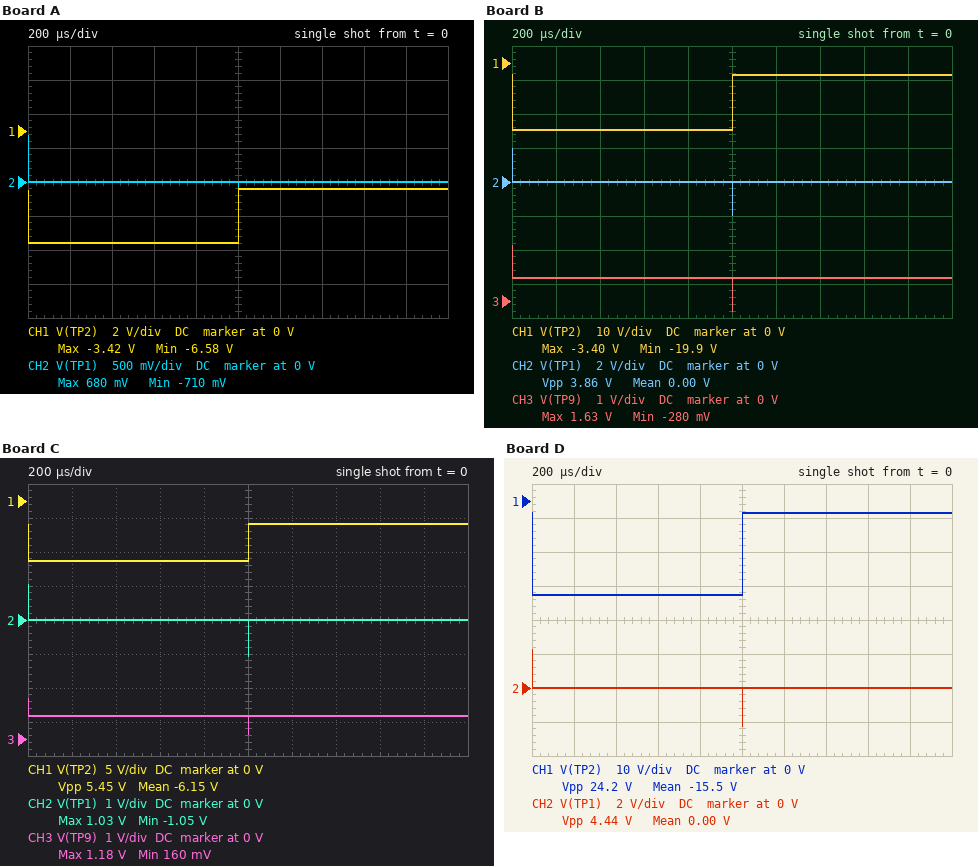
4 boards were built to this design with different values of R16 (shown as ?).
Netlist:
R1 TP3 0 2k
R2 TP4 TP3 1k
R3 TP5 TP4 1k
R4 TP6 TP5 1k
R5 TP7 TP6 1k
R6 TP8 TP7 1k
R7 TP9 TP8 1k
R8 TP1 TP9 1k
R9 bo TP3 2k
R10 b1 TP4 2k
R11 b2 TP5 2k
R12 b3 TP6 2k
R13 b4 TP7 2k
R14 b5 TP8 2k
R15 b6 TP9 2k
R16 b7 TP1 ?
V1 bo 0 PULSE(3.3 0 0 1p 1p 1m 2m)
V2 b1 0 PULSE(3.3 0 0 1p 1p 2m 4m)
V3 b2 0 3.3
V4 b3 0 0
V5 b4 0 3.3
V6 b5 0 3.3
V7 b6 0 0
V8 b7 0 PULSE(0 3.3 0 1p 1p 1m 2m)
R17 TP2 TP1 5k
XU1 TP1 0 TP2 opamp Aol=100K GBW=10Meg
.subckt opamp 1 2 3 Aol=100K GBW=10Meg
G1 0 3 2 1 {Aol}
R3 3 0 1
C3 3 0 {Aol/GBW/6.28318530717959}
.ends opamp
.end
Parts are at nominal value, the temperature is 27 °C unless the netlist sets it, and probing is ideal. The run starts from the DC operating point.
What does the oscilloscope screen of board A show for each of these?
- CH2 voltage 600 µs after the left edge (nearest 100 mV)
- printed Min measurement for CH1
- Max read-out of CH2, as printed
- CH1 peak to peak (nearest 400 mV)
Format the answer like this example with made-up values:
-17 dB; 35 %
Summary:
0 V; -6.58 V; 680 mV; 3.2 V
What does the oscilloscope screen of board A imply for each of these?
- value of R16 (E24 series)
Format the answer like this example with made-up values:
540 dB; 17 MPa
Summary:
5.1 kΩ
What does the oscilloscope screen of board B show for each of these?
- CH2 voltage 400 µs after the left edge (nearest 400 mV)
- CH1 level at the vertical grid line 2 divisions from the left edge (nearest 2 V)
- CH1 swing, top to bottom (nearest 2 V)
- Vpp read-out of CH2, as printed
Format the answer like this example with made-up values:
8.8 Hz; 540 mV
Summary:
0 V; -20 V; 16 V; 3.86 V
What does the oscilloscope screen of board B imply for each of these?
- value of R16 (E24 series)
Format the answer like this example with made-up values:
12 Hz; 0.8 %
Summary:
1 kΩ
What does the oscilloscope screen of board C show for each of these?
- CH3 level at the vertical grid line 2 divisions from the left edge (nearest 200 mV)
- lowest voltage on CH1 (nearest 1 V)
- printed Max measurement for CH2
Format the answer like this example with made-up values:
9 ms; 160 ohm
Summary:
600 mV; -9 V; 1.03 V
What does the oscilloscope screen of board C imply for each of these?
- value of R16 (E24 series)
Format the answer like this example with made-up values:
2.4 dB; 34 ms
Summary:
3 kΩ
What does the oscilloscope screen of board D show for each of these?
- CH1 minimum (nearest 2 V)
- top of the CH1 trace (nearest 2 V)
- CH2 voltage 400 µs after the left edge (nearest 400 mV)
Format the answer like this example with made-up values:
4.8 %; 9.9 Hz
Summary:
-28 V; -4 V; 0 V
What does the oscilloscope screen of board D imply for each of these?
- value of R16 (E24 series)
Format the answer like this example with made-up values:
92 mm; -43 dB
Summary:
680 Ω
